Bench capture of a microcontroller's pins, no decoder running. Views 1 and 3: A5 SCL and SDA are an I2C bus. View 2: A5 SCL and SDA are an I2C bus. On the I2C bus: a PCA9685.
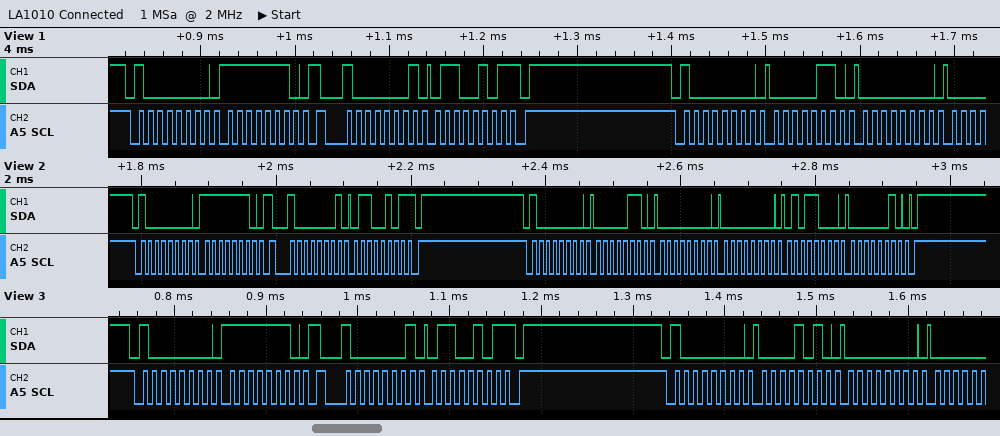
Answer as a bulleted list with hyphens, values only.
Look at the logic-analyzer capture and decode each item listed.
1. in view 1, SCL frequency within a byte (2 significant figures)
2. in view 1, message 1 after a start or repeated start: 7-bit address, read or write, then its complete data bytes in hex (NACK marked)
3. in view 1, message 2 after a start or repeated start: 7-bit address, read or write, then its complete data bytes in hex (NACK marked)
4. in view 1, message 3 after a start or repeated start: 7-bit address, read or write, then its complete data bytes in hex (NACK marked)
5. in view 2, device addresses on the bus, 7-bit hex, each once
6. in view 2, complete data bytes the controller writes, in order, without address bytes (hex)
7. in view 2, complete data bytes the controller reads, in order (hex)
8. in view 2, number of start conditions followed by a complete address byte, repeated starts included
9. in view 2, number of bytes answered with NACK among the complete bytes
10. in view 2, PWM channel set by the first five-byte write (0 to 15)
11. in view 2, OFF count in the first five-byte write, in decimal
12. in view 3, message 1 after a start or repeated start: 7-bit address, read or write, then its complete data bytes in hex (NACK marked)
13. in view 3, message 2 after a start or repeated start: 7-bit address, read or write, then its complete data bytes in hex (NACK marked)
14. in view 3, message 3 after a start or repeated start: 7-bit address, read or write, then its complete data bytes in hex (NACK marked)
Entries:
- 100 kHz
- 0x40 write: FE
- 0x40 read: 65 NACK
- 0x40 write: 06 00
- 0x40
- FE 06 00 00 58 02
- 65
- 3
- 1
- 0
- 600
- 0x40 write: FE
- 0x40 read: 65 NACK
- 0x40 write: 0A 00
